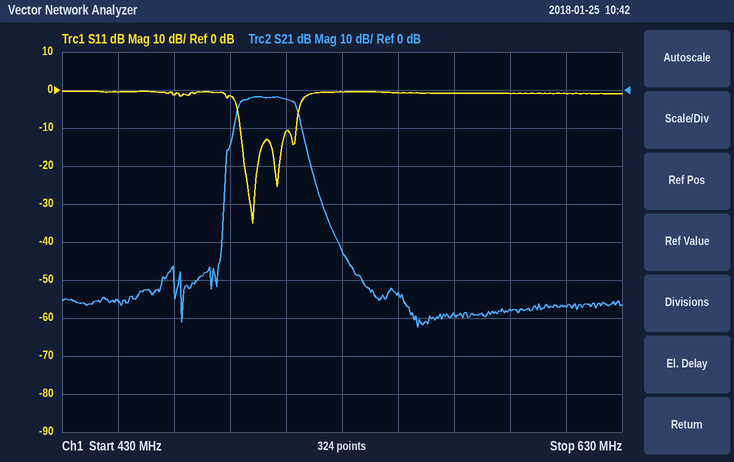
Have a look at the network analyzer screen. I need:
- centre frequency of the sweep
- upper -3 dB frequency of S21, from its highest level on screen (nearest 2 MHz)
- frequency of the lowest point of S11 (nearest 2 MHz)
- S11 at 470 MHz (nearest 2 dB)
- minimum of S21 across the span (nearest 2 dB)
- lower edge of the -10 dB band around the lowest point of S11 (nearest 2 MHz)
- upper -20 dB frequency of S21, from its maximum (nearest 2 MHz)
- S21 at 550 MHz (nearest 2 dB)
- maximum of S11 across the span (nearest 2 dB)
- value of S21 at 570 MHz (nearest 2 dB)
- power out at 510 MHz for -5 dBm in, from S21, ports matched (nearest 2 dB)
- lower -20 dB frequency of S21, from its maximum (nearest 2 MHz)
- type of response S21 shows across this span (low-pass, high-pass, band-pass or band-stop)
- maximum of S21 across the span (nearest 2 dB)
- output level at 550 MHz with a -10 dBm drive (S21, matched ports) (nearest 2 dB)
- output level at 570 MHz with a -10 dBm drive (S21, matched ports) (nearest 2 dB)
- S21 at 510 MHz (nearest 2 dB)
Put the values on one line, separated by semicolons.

530 MHz; 514 MHz; 498 MHz; -2 dB; -62 dB; 494 MHz; 520 MHz; -54 dB; 0 dB; -58 dB; -8 dBm; 488 MHz; band-pass; -2 dB; -64 dBm; -68 dBm; -2 dB
